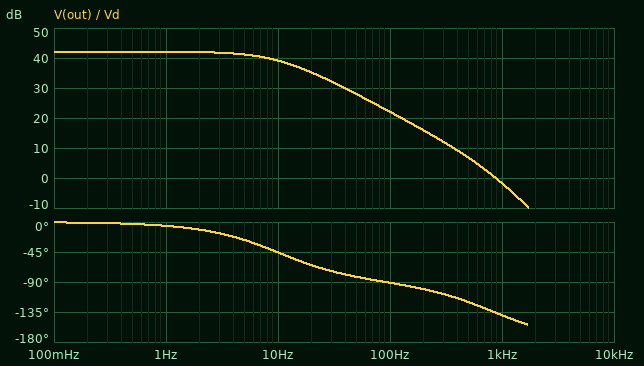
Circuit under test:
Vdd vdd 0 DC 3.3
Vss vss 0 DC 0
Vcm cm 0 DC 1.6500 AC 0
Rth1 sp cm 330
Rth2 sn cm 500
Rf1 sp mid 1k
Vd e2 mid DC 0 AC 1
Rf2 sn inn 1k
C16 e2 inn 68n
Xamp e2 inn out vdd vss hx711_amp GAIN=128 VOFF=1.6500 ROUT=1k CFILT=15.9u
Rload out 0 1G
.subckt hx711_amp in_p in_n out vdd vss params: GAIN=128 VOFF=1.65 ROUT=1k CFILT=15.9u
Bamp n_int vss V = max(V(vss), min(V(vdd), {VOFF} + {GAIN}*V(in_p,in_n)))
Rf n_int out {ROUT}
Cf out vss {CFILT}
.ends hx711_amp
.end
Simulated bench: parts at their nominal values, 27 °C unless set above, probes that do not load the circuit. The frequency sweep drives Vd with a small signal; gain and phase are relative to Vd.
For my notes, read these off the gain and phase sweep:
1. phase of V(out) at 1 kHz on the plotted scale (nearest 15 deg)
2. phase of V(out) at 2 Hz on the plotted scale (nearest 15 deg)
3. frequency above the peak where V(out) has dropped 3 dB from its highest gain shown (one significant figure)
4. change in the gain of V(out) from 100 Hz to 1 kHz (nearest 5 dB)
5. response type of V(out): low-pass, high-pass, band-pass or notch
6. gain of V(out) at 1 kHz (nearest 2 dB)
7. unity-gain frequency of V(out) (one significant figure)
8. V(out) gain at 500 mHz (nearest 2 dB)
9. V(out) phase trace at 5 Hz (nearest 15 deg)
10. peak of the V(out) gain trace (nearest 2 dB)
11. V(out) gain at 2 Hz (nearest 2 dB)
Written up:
-135 deg
-15 deg
10 Hz
-25 dB
low-pass
-2 dB
900 Hz
42 dB
-30 deg
42 dB
42 dB
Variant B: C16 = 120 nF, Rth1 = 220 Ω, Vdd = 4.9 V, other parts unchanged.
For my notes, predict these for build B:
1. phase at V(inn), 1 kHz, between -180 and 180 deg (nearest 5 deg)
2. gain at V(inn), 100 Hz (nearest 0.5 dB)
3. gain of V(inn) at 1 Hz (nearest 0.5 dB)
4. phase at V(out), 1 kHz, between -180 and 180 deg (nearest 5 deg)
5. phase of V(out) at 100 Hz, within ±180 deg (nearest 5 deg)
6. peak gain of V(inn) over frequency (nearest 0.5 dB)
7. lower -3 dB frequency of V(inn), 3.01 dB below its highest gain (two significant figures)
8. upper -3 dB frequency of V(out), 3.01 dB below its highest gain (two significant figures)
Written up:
25 deg
-19.0 dB
-59.0 dB
-155 deg
-95 deg
-5.0 dB
490 Hz
10 Hz
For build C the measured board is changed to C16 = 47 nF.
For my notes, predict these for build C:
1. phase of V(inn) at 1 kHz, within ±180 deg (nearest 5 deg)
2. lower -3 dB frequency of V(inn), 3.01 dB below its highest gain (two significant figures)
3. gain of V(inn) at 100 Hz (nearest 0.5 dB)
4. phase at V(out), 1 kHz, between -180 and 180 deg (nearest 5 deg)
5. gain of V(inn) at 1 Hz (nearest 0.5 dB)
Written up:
50 deg
1.2 kHz
-27.0 dB
-130 deg
-67.0 dB
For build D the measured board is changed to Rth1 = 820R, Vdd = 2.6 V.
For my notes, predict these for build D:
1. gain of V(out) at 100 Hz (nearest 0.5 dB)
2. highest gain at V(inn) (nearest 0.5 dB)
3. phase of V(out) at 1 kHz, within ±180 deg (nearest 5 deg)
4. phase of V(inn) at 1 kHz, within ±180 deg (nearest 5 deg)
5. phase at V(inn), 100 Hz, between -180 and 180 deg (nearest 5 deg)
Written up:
22.0 dB
-7.0 dB
-145 deg
35 deg
80 deg
